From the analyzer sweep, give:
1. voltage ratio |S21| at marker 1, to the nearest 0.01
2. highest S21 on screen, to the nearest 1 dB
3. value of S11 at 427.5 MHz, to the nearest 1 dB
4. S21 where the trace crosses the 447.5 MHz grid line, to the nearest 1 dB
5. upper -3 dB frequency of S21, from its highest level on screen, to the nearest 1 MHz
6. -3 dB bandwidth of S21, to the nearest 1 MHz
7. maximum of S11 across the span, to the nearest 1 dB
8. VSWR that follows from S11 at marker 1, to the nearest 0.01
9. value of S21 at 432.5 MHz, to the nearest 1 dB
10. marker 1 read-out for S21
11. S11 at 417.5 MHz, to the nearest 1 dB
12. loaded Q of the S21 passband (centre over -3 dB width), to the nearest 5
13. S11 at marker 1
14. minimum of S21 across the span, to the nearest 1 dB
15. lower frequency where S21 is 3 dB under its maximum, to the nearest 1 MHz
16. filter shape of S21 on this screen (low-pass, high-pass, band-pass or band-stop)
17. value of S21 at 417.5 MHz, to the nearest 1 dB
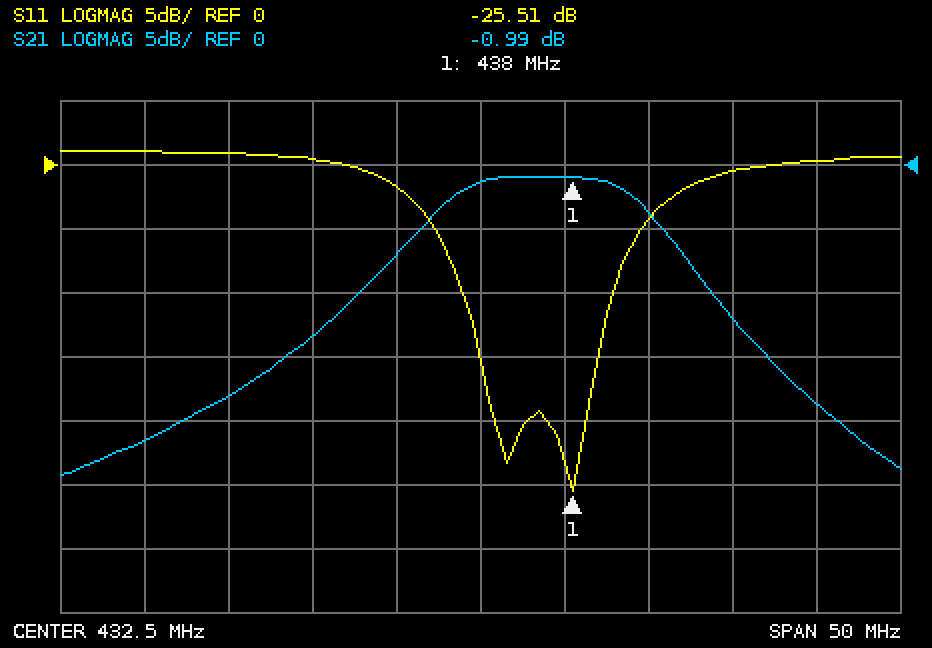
0.89
-1 dB
-2 dB
-12 dB
443 MHz
13 MHz
1 dB
1.11
-1 dB
-0.99 dB
1 dB
35
-25.51 dB
-24 dB
430 MHz
band-pass
-18 dB
